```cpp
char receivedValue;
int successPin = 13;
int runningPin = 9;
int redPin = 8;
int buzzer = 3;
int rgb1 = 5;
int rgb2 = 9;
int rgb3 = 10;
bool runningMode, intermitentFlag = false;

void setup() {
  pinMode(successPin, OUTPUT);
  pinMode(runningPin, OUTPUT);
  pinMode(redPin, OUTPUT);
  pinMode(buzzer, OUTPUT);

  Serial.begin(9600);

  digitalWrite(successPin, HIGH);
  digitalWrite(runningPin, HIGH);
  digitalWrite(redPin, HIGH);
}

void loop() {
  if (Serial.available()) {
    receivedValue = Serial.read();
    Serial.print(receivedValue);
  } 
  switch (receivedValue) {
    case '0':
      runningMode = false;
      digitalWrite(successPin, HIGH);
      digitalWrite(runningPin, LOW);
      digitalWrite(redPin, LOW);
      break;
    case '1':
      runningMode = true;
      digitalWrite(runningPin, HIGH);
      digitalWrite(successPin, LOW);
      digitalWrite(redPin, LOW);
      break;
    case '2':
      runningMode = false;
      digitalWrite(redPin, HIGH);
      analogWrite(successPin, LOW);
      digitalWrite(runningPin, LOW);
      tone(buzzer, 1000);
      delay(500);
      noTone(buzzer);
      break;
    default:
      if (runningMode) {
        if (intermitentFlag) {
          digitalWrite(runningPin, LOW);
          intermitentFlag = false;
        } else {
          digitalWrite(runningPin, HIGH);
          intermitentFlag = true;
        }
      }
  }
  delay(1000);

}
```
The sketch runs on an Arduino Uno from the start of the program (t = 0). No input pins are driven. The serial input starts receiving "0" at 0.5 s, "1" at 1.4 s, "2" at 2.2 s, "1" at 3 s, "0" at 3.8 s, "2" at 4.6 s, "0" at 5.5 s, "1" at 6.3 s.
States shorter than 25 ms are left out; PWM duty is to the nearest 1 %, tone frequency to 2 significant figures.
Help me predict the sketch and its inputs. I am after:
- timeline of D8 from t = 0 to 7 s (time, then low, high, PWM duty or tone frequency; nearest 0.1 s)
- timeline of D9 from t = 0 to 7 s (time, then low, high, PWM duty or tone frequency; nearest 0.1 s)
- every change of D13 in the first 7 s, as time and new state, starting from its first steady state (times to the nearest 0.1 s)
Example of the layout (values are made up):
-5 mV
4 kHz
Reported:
0 s high; 1 s low; 3 s high; 4.5 s low; 6.5 s high
0 s high; 1 s low; 2 s high; 3 s low; 4.5 s high; 5.5 s low
0 s high; 2 s low; 5.5 s high; 6.5 s low
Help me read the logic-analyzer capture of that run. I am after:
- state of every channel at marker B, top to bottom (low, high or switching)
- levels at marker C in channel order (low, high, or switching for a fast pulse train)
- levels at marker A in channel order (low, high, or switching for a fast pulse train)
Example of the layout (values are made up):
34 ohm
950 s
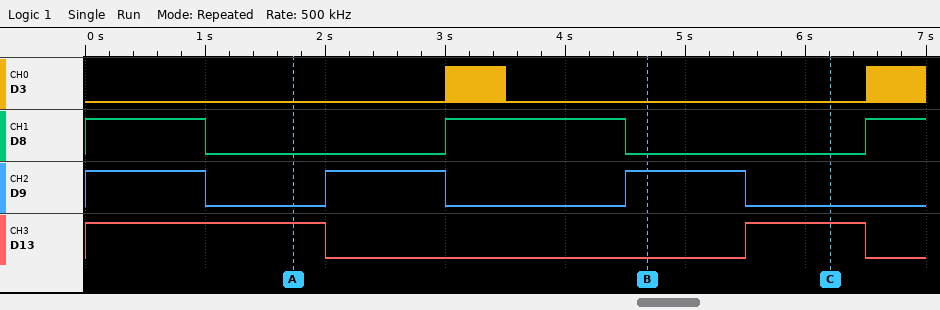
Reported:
D3 low, D8 low, D9 high, D13 low
D3 low, D8 low, D9 low, D13 high
D3 low, D8 low, D9 low, D13 high
